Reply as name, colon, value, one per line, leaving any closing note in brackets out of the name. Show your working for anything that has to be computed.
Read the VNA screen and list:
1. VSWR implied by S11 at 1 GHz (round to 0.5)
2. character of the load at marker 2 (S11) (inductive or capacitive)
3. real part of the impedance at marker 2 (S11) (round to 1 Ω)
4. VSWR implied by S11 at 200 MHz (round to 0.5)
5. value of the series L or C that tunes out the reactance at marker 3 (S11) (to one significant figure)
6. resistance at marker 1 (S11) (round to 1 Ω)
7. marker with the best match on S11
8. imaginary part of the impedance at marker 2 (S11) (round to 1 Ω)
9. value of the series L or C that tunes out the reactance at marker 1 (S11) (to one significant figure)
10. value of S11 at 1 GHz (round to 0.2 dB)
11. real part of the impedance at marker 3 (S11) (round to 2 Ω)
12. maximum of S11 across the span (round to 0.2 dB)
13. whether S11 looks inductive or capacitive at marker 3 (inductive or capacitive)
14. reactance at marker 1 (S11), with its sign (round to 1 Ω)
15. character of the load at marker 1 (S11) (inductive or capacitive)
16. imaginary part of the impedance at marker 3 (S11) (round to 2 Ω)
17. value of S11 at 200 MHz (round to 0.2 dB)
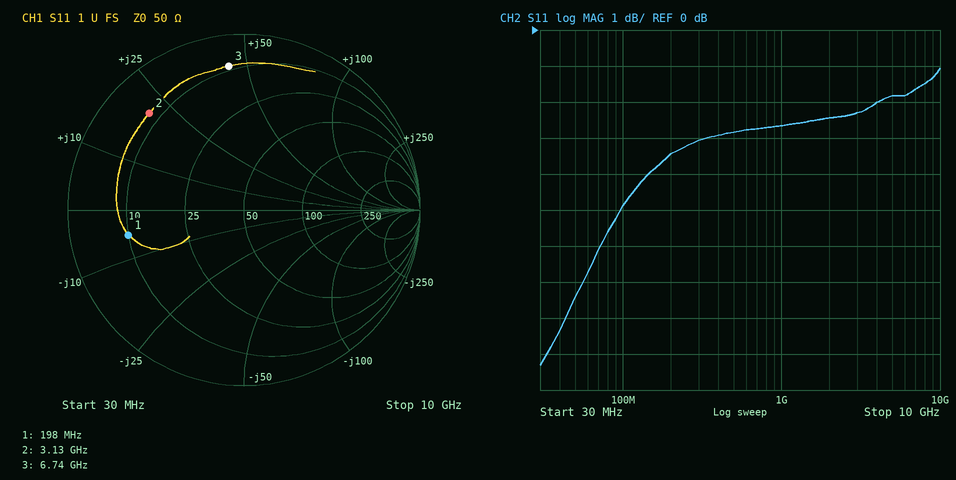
VSWR implied by S11 at 1 GHz: |Γ| = 10^(-2.6/20) = 0.7413; VSWR = (1 + 0.7413)/(1 − 0.7413) ≈ 6.73, so 6.5 to the nearest 0.5
character of the load at marker 2 (S11): inductive
real part of the impedance at marker 2 (S11): 8 Ω
VSWR implied by S11 at 200 MHz: |Γ| = 10^(-3.4/20) = 0.6761; VSWR = (1 + 0.6761)/(1 − 0.6761) ≈ 5.17, so 5.0 to the nearest 0.5
value of the series L or C that tunes out the reactance at marker 3 (S11): C = 1/(2π × 6.74 GHz × 44 Ω) ≈ 537 fF, so 500 fF to one significant figure
resistance at marker 1 (S11): 10 Ω
marker with the best match on S11: marker 1
imaginary part of the impedance at marker 2 (S11): +21 Ω
value of the series L or C that tunes out the reactance at marker 1 (S11): L = 5 Ω/(2π × 198 MHz) ≈ 4 nH
value of S11 at 1 GHz: -2.6 dB
real part of the impedance at marker 3 (S11): 8 Ω
maximum of S11 across the span: -1.0 dB
whether S11 looks inductive or capacitive at marker 3: inductive
reactance at marker 1 (S11), with its sign: -5 Ω
character of the load at marker 1 (S11): capacitive
imaginary part of the impedance at marker 3 (S11): +44 Ω
value of S11 at 200 MHz: -3.4 dB
